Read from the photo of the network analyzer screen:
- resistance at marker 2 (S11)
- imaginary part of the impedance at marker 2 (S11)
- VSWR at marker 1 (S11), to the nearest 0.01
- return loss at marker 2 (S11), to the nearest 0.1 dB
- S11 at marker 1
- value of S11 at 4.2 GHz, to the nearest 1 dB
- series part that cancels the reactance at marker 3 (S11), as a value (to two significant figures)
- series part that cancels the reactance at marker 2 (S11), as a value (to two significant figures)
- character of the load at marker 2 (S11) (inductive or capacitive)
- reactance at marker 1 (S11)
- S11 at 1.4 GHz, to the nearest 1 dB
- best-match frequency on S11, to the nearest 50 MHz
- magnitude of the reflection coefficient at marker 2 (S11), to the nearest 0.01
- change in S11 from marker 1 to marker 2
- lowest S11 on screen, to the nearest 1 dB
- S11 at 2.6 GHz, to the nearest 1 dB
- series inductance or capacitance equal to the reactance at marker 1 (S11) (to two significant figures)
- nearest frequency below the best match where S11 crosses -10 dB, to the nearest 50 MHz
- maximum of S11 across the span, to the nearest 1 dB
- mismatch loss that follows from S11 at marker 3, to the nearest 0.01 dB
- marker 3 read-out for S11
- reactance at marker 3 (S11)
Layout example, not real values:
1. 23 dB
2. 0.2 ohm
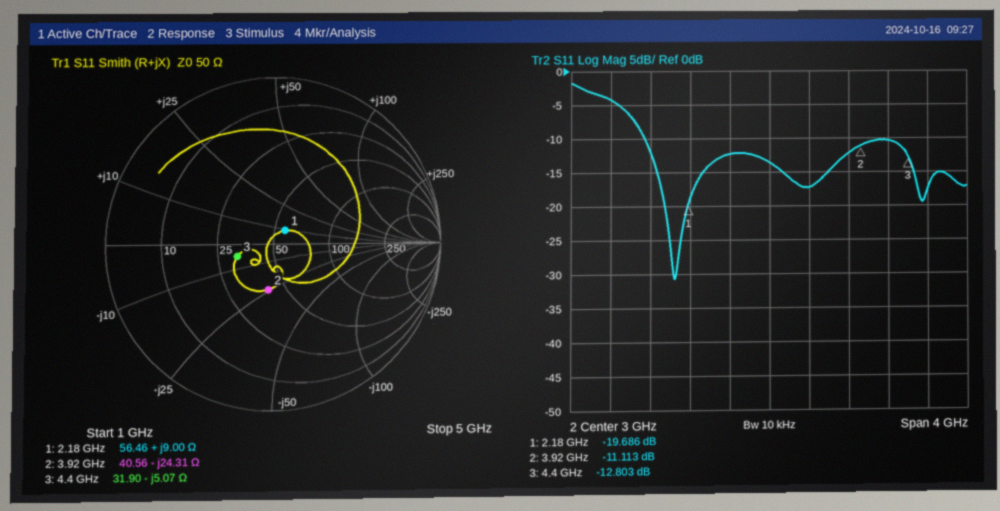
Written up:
1. 40.56 Ω
2. -24.31 Ω
3. 1.23
4. 11.1 dB
5. -19.686 dB
6. -10 dB
7. 180 pH
8. 990 pH
9. capacitive
10. +9.00 Ω
11. -4 dB
12. 2.05 GHz
13. 0.28
14. 8.573 dB
15. -31 dB
16. -12 dB
17. 660 pH
18. 1.75 GHz
19. -2 dB
20. 0.23 dB
21. -12.803 dB
22. -5.07 Ω
